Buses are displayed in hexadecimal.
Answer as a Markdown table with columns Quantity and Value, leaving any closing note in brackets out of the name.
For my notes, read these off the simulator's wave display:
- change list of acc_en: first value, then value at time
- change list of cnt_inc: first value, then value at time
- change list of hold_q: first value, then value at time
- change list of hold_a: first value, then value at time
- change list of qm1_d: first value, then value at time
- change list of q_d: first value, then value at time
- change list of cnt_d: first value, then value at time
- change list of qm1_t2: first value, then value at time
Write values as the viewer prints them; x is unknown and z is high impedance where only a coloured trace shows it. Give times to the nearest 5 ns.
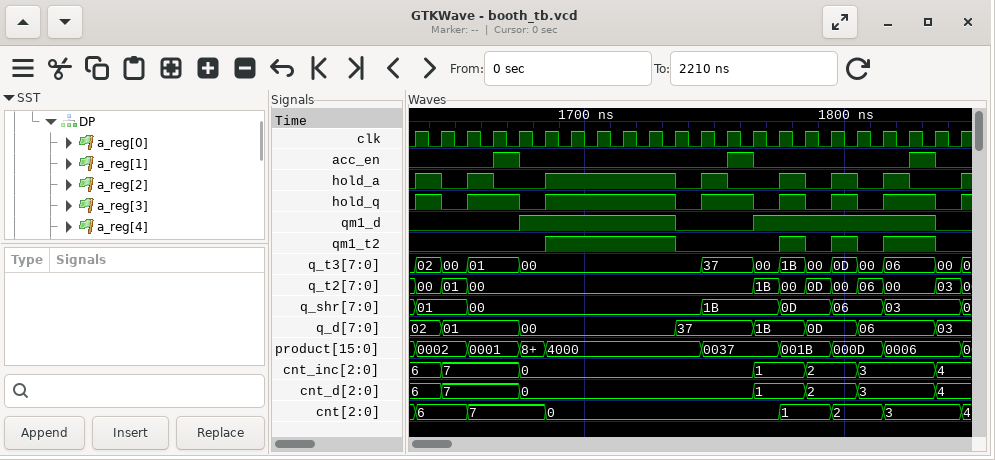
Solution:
| Quantity | Value |
|---|---|
| change list of acc_en: first value, then value at time | 0, 1 at 1665 ns, 0 at 1675 ns, 1 at 1755 ns, 0 at 1765 ns, 1 at 1825 ns, 0 at 1835 ns |
| change list of cnt_inc: first value, then value at time | 6, 7 at 1645 ns, 0 at 1675 ns, 1 at 1765 ns, 2 at 1785 ns, 3 at 1805 ns, 4 at 1835 ns |
| change list of hold_q: first value, then value at time | 0, 1 at 1635 ns, 0 at 1645 ns, 1 at 1655 ns, 0 at 1675 ns, 1 at 1685 ns, 0 at 1735 ns, 1 at 1745 ns, 0 at 1765 ns, 1 at 1775 ns, 0 at 1785 ns, 1 at 1795 ns, 0 at 1805 ns, 1 at 1815 ns, 0 at 1835 ns, 1 at 1845 ns |
| change list of hold_a: first value, then value at time | 0, 1 at 1635 ns, 0 at 1645 ns, 1 at 1655 ns, 0 at 1665 ns, 1 at 1685 ns, 0 at 1735 ns, 1 at 1745 ns, 0 at 1755 ns, 1 at 1775 ns, 0 at 1785 ns, 1 at 1795 ns, 0 at 1805 ns, 1 at 1815 ns, 0 at 1825 ns, 1 at 1845 ns |
| change list of qm1_d: first value, then value at time | 0, 1 at 1675 ns, 0 at 1735 ns, 1 at 1765 ns, 0 at 1835 ns |
| change list of q_d: first value, then value at time | 02, 01 at 1645 ns, 00 at 1675 ns, 37 at 1735 ns, 1B at 1765 ns, 0D at 1785 ns, 06 at 1805 ns, 03 at 1835 ns |
| change list of cnt_d: first value, then value at time | 6, 7 at 1645 ns, 0 at 1675 ns, 1 at 1765 ns, 2 at 1785 ns, 3 at 1805 ns, 4 at 1835 ns |
| change list of qm1_t2: first value, then value at time | 0, 1 at 1685 ns, 0 at 1735 ns, 1 at 1775 ns, 0 at 1785 ns, 1 at 1795 ns, 0 at 1805 ns, 1 at 1815 ns, 0 at 1835 ns |
